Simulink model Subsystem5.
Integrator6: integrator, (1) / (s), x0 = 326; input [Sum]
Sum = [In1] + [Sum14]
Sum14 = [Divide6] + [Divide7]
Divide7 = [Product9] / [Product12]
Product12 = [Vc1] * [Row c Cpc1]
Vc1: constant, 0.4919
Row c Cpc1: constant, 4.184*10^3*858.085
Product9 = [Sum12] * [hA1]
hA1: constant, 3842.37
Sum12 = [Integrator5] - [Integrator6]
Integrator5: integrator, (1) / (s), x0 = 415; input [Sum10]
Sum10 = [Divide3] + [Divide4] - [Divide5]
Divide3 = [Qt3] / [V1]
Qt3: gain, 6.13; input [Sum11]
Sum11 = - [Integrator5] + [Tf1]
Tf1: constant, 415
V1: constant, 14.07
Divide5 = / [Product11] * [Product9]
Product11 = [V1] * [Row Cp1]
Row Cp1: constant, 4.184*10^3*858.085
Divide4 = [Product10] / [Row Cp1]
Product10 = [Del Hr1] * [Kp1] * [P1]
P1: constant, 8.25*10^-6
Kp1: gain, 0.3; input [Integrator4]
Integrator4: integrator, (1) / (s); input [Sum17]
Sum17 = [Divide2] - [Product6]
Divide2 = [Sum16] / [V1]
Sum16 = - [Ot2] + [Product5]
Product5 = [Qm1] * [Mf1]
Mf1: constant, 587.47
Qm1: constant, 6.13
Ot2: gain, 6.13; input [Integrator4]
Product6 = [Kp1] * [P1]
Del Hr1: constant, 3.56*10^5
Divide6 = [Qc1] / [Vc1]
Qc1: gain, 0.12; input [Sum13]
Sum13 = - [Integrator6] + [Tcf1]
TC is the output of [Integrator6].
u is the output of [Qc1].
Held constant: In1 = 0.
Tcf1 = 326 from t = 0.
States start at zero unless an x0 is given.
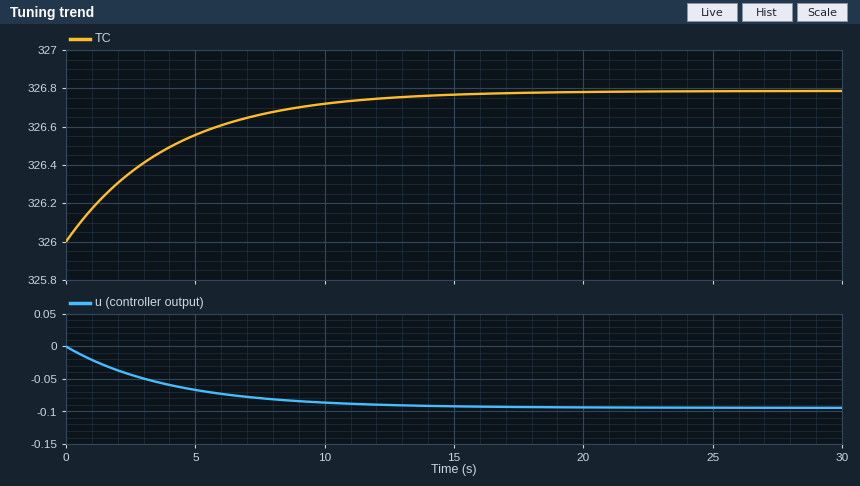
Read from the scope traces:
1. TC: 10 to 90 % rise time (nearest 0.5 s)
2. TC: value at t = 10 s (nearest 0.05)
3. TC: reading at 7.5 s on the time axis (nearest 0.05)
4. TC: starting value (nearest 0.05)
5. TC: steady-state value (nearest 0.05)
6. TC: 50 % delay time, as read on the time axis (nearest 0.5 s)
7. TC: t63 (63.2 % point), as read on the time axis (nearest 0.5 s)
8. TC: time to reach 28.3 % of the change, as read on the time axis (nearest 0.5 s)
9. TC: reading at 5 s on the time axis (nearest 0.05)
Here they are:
9.0 s
326.70
326.65
326.00
326.80
3.0 s
4.0 s
1.5 s
326.55
